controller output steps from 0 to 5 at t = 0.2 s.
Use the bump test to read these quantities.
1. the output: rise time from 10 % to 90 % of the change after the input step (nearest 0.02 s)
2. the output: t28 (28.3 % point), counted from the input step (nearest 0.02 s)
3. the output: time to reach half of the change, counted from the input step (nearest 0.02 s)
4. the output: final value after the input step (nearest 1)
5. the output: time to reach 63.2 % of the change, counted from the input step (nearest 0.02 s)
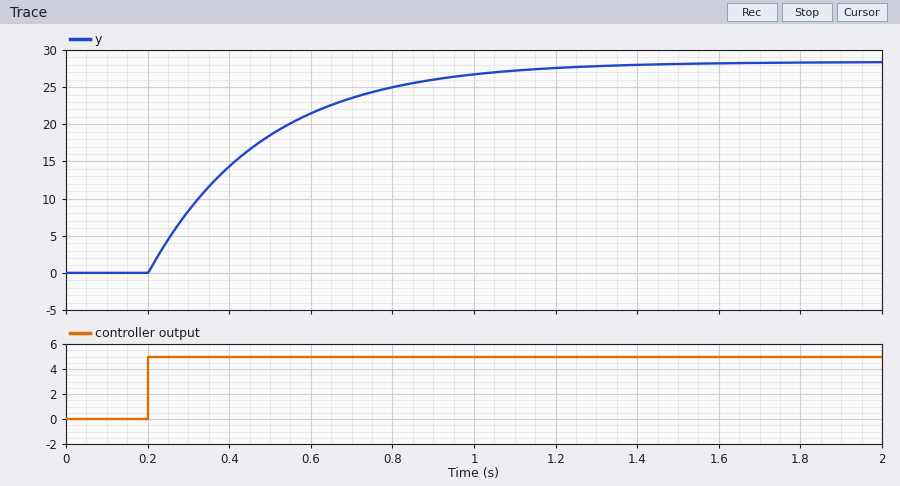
0.62 s
0.10 s
0.20 s
28
0.28 s
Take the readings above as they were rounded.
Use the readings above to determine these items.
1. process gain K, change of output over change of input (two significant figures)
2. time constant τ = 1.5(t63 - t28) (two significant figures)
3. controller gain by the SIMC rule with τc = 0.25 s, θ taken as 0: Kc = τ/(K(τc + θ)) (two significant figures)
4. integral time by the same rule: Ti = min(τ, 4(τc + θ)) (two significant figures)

5.6
0.27 s
0.19
0.27 s
